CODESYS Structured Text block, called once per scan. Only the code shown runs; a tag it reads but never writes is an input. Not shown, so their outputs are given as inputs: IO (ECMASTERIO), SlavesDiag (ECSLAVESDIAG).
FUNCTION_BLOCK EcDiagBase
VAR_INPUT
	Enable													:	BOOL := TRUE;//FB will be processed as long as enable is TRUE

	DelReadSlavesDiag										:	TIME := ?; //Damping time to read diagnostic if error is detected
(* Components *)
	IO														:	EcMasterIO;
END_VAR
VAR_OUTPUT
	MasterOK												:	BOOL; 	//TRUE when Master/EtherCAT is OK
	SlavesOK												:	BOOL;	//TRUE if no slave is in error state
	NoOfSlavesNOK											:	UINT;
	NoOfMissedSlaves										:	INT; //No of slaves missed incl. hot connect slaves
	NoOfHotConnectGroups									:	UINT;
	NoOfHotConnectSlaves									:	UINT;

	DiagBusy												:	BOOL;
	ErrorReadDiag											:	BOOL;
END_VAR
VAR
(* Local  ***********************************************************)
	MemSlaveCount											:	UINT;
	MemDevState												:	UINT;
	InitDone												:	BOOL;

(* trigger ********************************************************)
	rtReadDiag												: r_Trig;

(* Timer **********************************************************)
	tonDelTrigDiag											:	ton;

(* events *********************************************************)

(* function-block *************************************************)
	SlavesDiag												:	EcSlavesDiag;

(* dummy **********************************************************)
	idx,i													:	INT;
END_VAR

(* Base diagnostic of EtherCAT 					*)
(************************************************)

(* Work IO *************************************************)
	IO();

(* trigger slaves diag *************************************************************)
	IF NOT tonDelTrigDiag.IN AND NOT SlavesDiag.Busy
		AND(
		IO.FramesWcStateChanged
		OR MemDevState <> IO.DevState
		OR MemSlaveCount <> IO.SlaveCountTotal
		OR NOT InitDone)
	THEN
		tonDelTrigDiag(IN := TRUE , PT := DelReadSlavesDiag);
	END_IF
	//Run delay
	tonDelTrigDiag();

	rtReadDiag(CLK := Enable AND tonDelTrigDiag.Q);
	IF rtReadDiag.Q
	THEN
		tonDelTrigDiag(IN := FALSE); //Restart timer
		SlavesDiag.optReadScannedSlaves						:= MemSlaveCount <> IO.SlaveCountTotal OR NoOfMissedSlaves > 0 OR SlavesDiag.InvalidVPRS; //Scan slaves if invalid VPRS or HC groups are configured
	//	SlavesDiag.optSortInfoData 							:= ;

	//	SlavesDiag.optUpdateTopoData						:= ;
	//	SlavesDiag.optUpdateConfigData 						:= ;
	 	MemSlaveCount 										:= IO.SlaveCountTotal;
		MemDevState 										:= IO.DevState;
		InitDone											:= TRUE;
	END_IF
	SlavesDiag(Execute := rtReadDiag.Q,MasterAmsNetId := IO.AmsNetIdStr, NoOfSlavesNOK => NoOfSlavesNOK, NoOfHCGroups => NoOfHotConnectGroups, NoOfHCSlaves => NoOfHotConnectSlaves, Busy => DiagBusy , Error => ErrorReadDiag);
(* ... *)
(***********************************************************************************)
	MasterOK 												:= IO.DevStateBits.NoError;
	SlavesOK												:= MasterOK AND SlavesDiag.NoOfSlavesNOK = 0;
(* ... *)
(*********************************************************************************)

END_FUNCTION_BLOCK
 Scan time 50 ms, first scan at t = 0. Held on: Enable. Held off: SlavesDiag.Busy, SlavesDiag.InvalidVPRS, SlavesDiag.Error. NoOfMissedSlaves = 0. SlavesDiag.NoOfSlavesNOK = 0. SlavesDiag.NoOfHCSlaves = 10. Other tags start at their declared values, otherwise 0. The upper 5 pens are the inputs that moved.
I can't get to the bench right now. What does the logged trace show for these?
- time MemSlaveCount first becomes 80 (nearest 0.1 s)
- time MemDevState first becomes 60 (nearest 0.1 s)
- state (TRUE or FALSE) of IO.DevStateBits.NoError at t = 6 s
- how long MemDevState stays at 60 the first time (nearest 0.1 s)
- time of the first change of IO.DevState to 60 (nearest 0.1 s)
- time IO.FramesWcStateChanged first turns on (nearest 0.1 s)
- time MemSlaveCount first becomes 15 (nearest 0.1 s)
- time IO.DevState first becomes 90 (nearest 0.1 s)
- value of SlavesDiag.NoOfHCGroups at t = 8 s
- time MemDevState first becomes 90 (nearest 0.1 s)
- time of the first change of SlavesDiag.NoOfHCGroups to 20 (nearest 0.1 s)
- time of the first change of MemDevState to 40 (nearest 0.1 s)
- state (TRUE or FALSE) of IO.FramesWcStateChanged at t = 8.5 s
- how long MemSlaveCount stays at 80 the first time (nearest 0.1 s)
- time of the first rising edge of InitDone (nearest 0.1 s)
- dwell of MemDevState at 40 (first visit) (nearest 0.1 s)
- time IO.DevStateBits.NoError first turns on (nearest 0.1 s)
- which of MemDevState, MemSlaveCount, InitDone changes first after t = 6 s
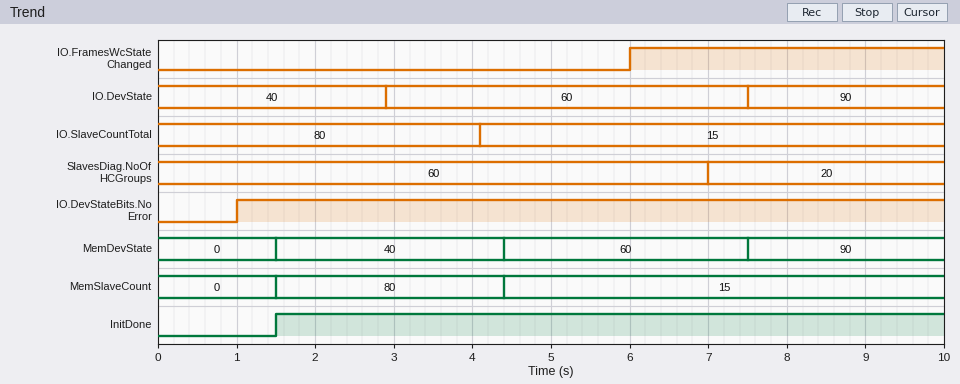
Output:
1.5 s
4.4 s
TRUE
3.1 s
2.9 s
6.0 s
4.4 s
7.5 s
20
7.5 s
7.0 s
1.5 s
TRUE
2.9 s
1.5 s
2.9 s
1.0 s
MemDevState
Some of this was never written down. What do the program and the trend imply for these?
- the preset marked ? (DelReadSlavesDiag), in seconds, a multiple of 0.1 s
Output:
1.5 s
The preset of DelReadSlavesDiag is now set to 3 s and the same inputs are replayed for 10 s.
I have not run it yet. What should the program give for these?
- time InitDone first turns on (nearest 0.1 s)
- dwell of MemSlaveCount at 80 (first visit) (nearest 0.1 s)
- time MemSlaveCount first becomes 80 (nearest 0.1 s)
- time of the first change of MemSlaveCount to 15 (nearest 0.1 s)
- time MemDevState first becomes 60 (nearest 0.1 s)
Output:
3.0 s
4.1 s
3.0 s
7.1 s
3.0 s
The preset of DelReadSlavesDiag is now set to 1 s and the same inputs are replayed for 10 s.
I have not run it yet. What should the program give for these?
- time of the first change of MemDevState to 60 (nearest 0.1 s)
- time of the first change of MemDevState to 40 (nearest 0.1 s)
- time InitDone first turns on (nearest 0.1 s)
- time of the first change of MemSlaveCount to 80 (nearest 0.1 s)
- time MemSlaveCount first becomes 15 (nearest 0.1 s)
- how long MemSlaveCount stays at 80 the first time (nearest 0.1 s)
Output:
3.9 s
1.0 s
1.0 s
1.0 s
5.1 s
4.1 s
